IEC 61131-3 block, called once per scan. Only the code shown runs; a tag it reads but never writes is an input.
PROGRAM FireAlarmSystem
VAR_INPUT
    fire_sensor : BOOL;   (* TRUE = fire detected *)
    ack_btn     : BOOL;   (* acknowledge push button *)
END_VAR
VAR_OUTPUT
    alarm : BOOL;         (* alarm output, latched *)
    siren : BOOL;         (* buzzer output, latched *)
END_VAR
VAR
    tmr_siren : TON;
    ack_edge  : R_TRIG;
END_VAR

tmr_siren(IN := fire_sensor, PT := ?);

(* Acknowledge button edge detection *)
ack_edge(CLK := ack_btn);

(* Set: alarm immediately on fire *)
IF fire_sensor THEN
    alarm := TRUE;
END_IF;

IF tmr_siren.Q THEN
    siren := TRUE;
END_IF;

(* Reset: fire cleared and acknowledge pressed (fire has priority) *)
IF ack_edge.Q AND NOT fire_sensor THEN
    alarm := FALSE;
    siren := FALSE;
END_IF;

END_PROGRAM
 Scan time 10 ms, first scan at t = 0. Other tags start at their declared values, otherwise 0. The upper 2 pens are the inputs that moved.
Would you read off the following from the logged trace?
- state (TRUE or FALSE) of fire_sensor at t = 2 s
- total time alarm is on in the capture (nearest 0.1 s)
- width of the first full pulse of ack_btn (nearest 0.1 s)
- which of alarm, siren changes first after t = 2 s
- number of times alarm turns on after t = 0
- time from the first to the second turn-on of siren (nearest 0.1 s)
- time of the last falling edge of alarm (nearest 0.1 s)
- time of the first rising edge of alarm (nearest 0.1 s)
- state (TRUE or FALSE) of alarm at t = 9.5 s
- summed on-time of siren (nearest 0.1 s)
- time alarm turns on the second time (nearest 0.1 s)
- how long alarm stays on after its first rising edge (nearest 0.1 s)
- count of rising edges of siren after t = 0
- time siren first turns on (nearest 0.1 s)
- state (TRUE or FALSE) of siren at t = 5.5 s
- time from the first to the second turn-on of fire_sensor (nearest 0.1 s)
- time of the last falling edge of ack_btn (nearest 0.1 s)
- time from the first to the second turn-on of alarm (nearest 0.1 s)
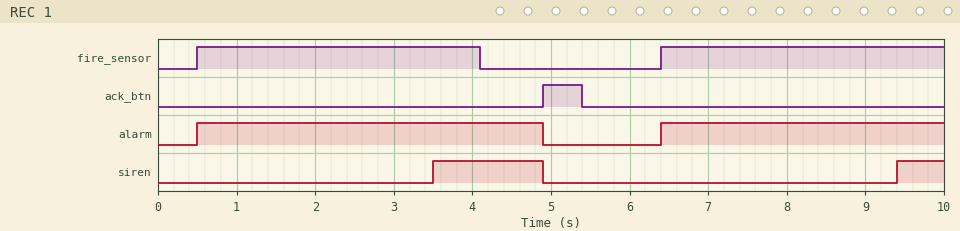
TRUE
8.0 s
0.5 s
siren
2
5.9 s
4.9 s
0.5 s
TRUE
2.0 s
6.4 s
4.4 s
2
3.5 s
FALSE
5.9 s
5.4 s
5.9 s
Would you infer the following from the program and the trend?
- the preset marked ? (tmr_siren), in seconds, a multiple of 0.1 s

3.0 s
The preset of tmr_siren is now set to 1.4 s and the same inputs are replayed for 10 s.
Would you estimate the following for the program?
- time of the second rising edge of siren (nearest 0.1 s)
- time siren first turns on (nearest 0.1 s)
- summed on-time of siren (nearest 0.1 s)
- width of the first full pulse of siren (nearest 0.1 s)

7.8 s
1.9 s
5.2 s
3.0 s
